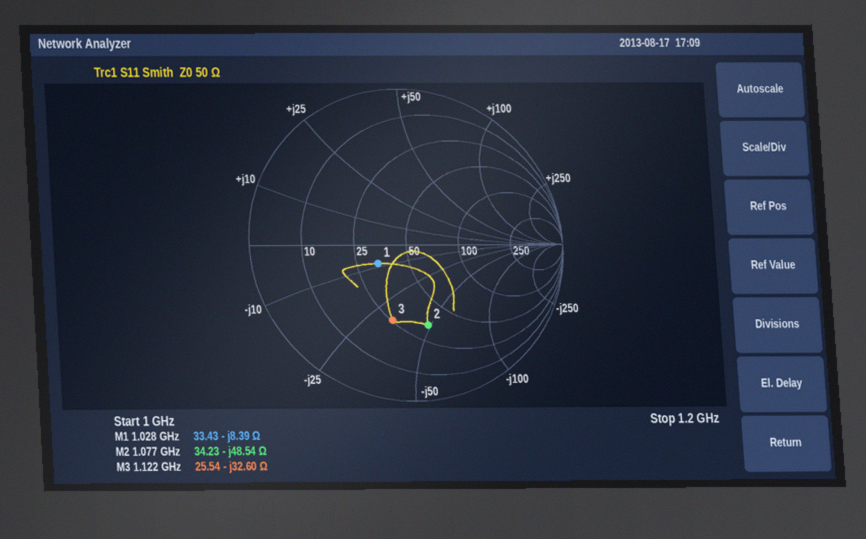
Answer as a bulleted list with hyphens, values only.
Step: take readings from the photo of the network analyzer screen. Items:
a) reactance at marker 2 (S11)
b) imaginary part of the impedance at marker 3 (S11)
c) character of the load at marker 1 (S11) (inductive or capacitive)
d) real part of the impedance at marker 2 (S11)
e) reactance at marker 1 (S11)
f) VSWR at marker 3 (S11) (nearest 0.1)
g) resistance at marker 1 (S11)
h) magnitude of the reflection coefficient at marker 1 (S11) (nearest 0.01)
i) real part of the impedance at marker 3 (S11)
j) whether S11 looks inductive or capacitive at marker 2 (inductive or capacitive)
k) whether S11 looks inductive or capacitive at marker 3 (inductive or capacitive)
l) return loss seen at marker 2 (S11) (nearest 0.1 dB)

- -48.54 Ω
- -32.60 Ω
- capacitive
- 34.23 Ω
- -8.39 Ω
- 3.0
- 33.43 Ω
- 0.22
- 25.54 Ω
- capacitive
- capacitive
- 5.6 dB
